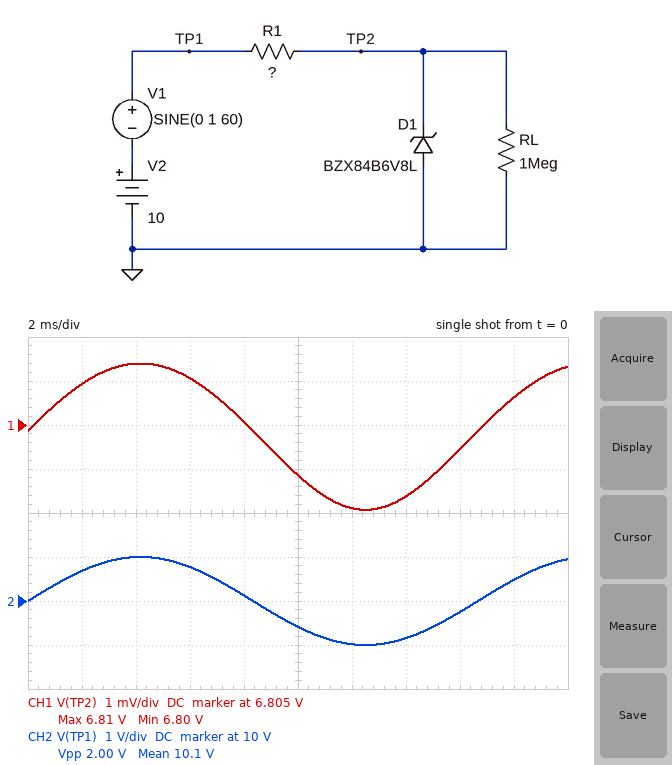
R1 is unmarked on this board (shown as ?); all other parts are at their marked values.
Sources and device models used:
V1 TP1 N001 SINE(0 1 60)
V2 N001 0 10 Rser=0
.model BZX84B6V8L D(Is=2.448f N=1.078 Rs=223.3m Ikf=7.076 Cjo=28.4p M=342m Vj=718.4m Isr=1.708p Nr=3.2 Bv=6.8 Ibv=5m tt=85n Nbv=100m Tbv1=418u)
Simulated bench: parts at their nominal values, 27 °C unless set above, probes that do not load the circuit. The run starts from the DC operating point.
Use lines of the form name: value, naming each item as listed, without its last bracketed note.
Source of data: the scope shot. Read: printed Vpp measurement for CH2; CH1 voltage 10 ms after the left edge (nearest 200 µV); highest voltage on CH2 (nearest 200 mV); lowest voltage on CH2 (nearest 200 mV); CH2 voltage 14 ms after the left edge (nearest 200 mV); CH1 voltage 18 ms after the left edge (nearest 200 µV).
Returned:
printed Vpp measurement for CH2: 2.00 V
CH1 voltage 10 ms after the left edge: 6.8038 V
highest voltage on CH2: 11.0 V
lowest voltage on CH2: 9.0 V
CH2 voltage 14 ms after the left edge: 9.2 V
CH1 voltage 18 ms after the left edge: 6.8056 V
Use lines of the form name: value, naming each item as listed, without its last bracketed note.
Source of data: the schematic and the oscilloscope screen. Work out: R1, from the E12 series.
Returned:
R1, from the E12 series: 270 Ω
